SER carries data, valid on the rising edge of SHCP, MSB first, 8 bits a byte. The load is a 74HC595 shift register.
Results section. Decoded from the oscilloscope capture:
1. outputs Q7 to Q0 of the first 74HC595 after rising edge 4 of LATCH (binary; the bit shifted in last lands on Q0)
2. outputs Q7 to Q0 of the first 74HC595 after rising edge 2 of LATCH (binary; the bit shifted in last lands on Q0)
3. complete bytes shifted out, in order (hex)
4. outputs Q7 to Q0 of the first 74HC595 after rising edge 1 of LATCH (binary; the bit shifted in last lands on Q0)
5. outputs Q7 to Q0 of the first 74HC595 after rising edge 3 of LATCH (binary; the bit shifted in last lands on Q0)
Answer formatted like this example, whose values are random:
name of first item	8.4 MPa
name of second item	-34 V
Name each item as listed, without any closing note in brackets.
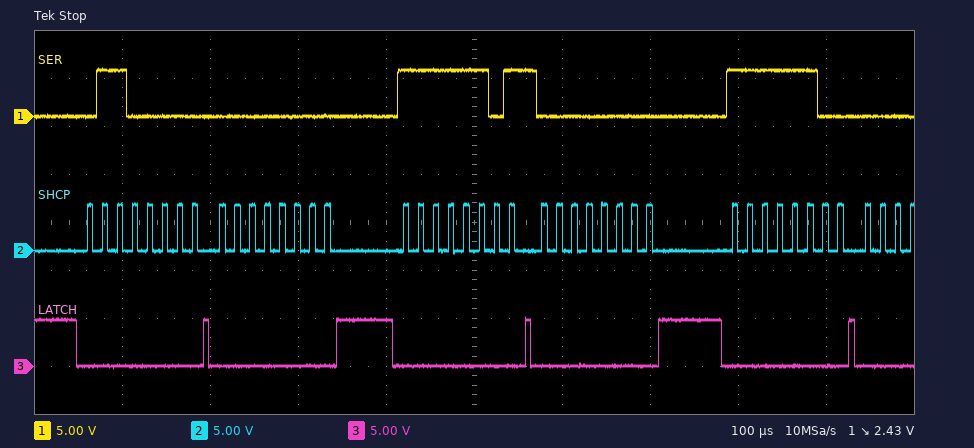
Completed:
outputs Q7 to Q0 of the first 74HC595 after rising edge 4 of LATCH	00000000
outputs Q7 to Q0 of the first 74HC595 after rising edge 2 of LATCH	00000000
complete bytes shifted out, in order	60 00 FD 00 FC
outputs Q7 to Q0 of the first 74HC595 after rising edge 1 of LATCH	01100000
outputs Q7 to Q0 of the first 74HC595 after rising edge 3 of LATCH	11111101
